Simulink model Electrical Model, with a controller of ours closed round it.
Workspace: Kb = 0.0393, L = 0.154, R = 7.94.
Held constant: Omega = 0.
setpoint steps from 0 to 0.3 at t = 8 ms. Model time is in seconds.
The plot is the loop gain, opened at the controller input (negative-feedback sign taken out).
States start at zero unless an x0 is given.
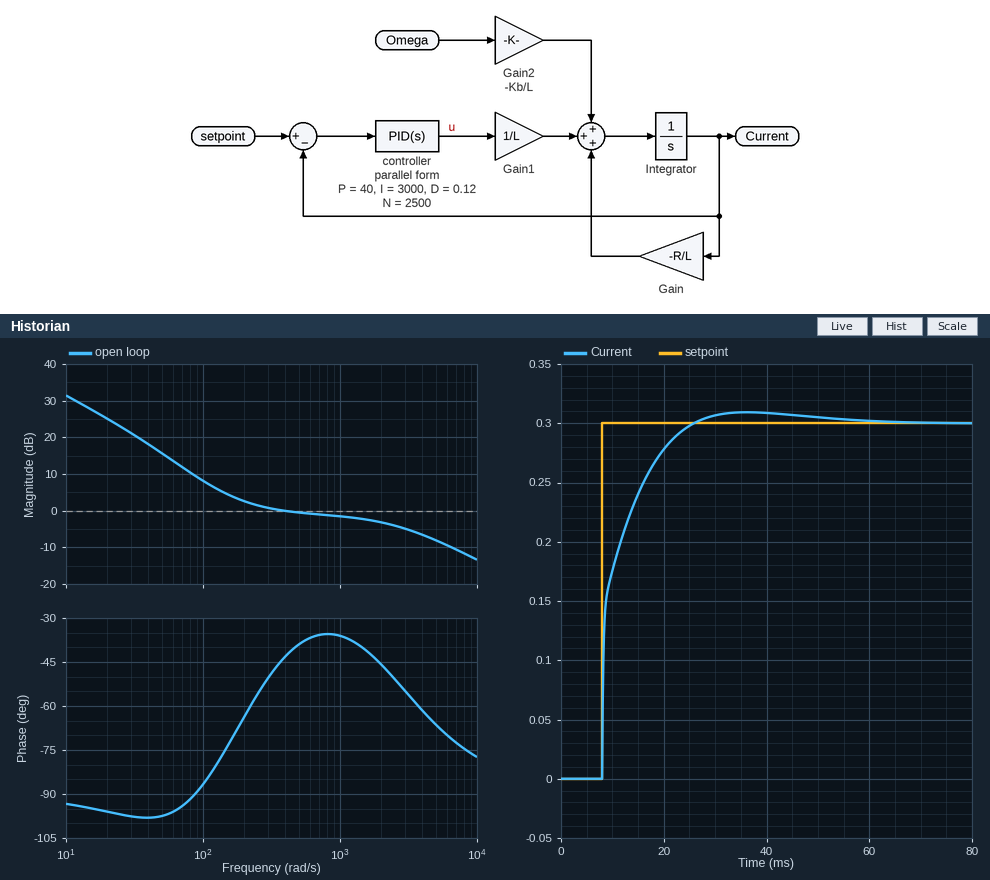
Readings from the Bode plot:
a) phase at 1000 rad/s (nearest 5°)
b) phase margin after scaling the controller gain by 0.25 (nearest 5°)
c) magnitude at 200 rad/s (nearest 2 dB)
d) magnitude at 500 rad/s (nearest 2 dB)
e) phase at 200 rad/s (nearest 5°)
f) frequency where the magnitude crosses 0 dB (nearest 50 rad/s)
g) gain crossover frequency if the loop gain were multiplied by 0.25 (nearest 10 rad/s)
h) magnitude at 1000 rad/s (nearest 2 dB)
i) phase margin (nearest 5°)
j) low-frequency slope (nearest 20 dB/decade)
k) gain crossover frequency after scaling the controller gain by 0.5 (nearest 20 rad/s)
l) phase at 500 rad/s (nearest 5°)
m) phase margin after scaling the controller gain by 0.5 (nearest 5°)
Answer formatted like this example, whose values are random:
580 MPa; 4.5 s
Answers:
-35°; 85°; 2 dB; 0 dB; -65°; 400 rad/s; 70 rad/s; -2 dB; 135°; -20 dB/decade; 120 rad/s; -40°; 100°
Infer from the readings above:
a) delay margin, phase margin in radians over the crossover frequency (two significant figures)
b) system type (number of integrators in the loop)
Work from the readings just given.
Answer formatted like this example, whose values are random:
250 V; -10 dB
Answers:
0.0059 s; 1
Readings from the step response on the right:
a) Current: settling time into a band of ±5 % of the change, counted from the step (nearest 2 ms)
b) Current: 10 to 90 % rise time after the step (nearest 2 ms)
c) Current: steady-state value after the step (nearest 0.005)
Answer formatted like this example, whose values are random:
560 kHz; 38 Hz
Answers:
14 ms; 10 ms; 0.300
